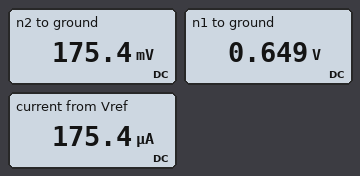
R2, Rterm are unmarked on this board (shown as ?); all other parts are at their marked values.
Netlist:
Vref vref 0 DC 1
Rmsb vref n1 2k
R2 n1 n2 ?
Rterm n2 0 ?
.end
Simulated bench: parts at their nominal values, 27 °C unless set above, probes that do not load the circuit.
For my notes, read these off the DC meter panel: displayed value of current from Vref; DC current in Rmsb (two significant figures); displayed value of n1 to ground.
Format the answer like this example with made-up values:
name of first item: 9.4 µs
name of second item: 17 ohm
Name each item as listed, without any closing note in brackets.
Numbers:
displayed value of current from Vref: 175.4 µA
DC current in Rmsb: 180 µA
displayed value of n1 to ground: 0.649 V
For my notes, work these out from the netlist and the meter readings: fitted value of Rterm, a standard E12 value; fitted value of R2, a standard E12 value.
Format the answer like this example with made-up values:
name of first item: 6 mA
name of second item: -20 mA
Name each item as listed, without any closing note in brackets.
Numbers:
fitted value of Rterm, a standard E12 value: 1 kΩ
fitted value of R2, a standard E12 value: 2.7 kΩ
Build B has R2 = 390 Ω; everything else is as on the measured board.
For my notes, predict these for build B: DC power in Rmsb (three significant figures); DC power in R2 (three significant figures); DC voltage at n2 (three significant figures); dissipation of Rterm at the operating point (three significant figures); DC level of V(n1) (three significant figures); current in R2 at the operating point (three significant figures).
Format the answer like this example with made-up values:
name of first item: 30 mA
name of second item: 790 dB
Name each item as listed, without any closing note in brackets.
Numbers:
DC power in Rmsb: 174 µW
DC power in R2: 33.9 µW
DC voltage at n2: 295 mV
dissipation of Rterm at the operating point: 87.0 µW
DC level of V(n1): 410 mV
current in R2 at the operating point: 295 µA
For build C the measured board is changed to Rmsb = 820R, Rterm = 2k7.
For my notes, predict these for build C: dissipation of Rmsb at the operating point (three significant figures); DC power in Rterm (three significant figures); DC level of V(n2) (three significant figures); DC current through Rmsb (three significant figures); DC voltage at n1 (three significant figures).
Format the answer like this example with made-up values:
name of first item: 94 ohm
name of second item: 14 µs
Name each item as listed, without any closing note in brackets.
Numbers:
dissipation of Rmsb at the operating point: 21.2 µW
DC power in Rterm: 69.8 µW
DC level of V(n2): 434 mV
DC current through Rmsb: 161 µA
DC voltage at n1: 868 mV
